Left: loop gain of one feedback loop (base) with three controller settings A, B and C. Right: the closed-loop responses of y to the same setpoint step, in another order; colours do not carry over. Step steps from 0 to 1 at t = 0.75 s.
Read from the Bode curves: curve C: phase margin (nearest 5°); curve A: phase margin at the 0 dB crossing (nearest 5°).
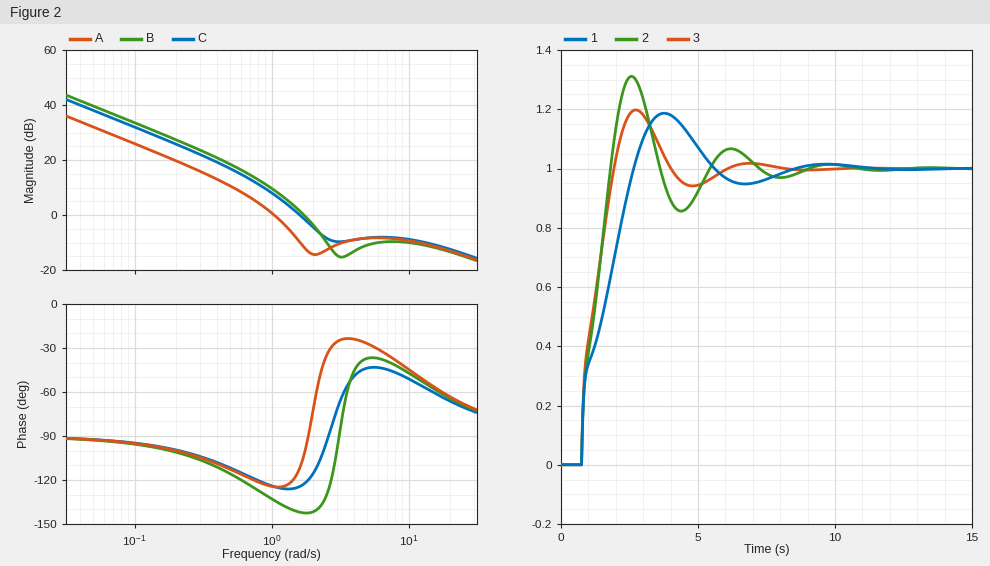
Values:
55°
55°
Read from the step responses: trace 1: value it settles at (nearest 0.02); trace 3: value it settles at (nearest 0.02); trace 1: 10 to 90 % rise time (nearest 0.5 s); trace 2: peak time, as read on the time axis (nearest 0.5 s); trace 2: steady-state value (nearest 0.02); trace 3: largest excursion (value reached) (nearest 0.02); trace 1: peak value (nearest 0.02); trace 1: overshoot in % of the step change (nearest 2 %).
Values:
1.00
1.00
1.5 s
2.5 s
1.00
1.20
1.18
18 %
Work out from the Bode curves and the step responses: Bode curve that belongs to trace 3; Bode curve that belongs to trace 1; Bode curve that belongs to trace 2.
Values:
C
A
B
